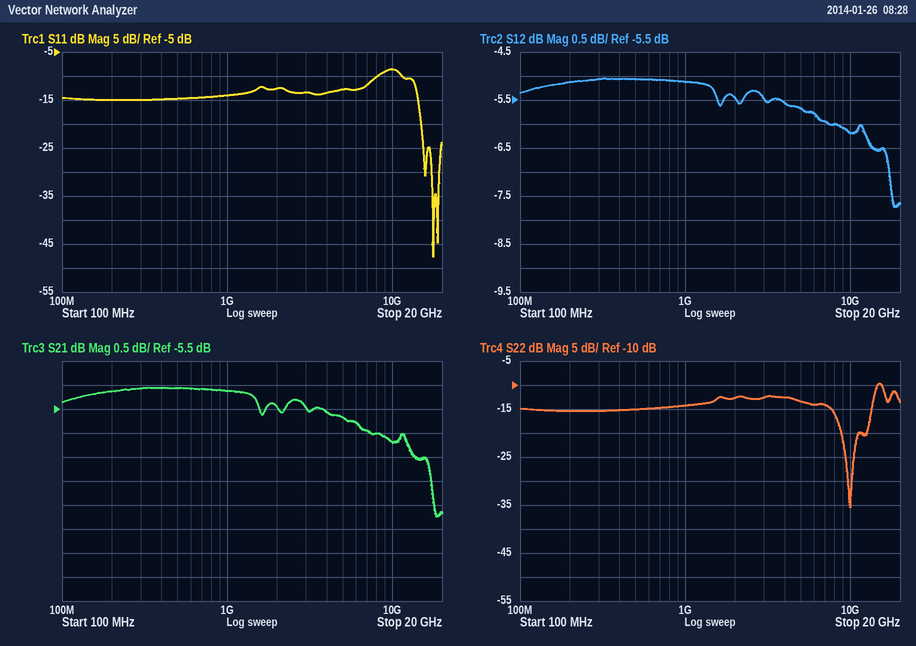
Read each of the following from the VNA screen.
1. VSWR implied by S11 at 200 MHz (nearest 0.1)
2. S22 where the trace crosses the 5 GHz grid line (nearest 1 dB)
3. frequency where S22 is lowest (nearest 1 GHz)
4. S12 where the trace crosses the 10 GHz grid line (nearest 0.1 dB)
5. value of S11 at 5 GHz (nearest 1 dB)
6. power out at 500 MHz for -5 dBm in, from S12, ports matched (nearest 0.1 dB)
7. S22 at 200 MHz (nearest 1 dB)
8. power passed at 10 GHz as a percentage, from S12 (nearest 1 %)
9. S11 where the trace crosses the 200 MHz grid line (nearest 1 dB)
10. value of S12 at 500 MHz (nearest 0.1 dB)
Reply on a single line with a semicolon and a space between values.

1.4; -13 dB; 10 GHz; -6.2 dB; -13 dB; -10.1 dBm; -15 dB; 24 %; -15 dB; -5.1 dB
